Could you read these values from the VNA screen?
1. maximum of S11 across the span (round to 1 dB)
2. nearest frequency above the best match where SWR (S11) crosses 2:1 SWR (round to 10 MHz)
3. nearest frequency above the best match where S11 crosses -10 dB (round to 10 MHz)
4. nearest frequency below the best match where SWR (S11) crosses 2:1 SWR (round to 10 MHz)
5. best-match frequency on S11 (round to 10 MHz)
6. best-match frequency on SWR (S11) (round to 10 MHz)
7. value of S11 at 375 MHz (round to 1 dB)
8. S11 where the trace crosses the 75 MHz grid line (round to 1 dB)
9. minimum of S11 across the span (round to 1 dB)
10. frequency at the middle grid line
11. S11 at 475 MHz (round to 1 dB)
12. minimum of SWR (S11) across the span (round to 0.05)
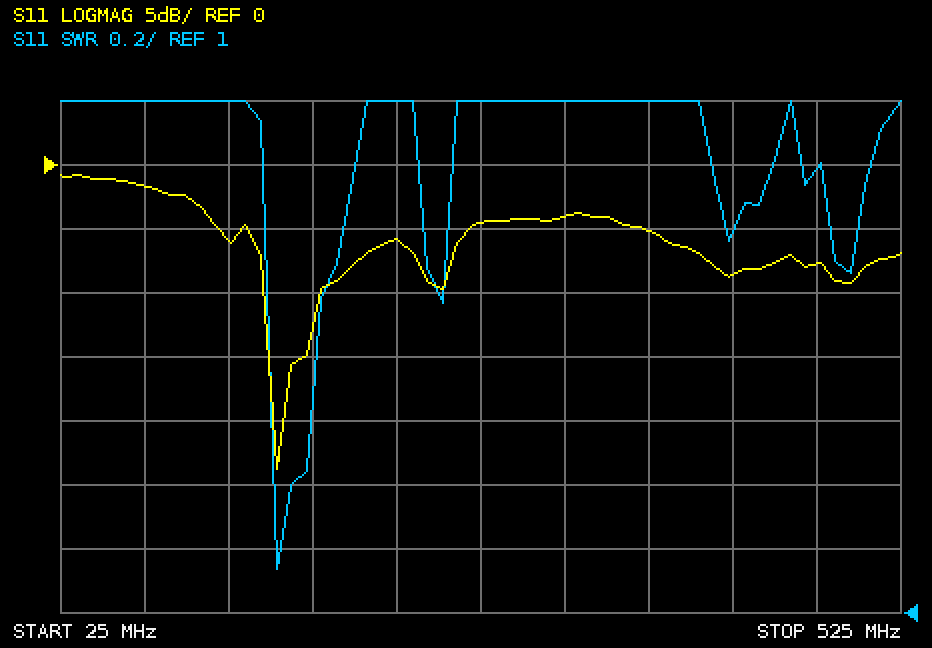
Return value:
-1 dB
180 MHz
180 MHz
150 MHz
150 MHz
150 MHz
-5 dB
-2 dB
-24 dB
275 MHz
-8 dB
1.15
